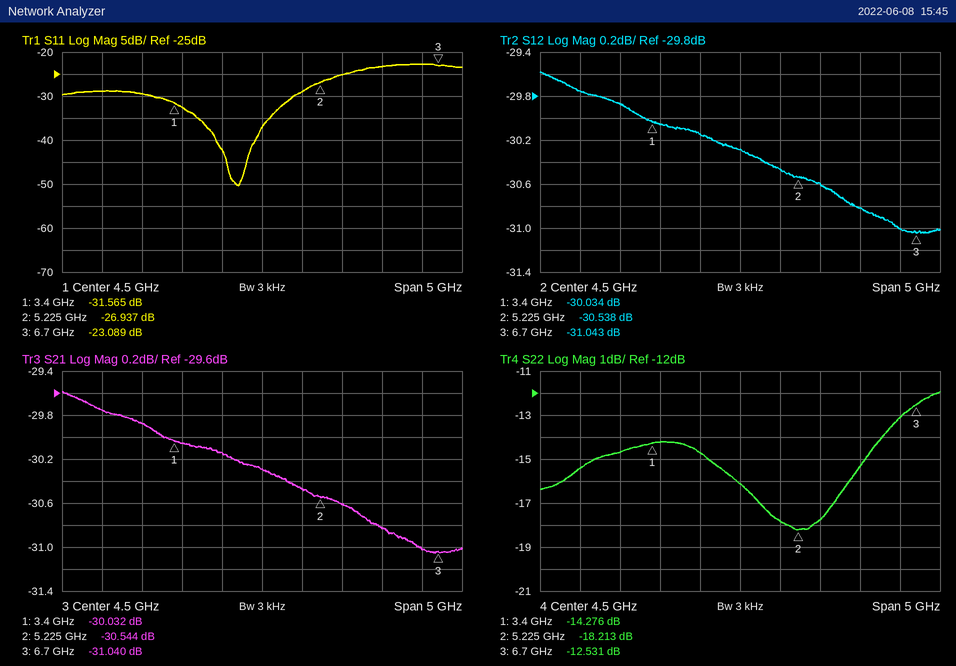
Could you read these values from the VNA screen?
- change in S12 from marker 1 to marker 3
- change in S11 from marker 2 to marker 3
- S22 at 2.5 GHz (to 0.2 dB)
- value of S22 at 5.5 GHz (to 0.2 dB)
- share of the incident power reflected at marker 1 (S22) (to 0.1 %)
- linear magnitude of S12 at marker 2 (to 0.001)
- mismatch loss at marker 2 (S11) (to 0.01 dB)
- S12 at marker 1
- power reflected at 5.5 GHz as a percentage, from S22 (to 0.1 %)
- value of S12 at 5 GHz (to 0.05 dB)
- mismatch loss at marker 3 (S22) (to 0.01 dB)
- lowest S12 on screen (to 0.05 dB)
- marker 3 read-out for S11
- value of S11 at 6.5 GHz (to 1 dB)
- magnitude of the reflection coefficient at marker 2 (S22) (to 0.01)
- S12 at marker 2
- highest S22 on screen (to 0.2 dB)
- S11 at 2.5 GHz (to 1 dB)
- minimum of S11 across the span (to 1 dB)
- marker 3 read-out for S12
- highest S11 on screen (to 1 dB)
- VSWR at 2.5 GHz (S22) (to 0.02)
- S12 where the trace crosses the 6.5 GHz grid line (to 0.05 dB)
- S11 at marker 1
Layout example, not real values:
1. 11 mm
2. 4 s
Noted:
1. -1.009 dB
2. 3.848 dB
3. -15.4 dB
4. -17.8 dB
5. 3.7 %
6. 0.030
7. 0.01 dB
8. -30.034 dB
9. 1.7 %
10. -30.45 dB
11. 0.25 dB
12. -31.05 dB
13. -23.089 dB
14. -23 dB
15. 0.12
16. -30.538 dB
17. -12.0 dB
18. -29 dB
19. -50 dB
20. -31.043 dB
21. -23 dB
22. 1.40
23. -31.00 dB
24. -31.565 dB
